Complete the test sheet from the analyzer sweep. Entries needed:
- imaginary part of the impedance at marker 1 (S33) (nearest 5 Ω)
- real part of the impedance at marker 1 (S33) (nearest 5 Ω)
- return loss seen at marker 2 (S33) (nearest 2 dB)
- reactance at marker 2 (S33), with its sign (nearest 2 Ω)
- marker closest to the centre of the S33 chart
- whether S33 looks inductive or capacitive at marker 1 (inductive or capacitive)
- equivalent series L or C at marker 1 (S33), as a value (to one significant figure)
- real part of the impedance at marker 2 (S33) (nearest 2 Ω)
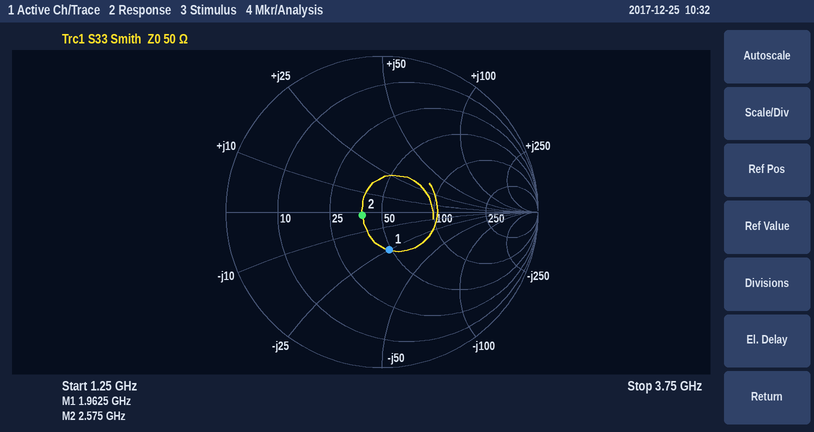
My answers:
-25 Ω
50 Ω
18 dB
-2 Ω
marker 2
capacitive
3 pF
38 Ω
